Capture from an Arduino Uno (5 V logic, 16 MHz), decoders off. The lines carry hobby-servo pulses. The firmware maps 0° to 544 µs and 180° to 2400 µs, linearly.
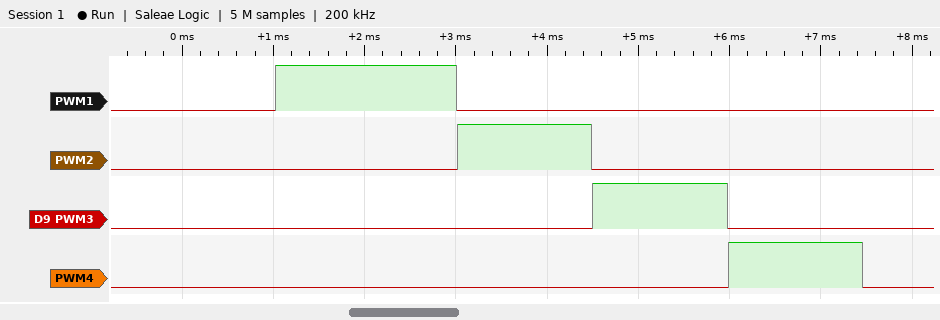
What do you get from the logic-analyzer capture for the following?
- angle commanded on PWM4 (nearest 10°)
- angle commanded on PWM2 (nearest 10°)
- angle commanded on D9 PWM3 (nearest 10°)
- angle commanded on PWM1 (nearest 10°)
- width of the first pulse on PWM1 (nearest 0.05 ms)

90°
90°
90°
140°
2.00 ms
